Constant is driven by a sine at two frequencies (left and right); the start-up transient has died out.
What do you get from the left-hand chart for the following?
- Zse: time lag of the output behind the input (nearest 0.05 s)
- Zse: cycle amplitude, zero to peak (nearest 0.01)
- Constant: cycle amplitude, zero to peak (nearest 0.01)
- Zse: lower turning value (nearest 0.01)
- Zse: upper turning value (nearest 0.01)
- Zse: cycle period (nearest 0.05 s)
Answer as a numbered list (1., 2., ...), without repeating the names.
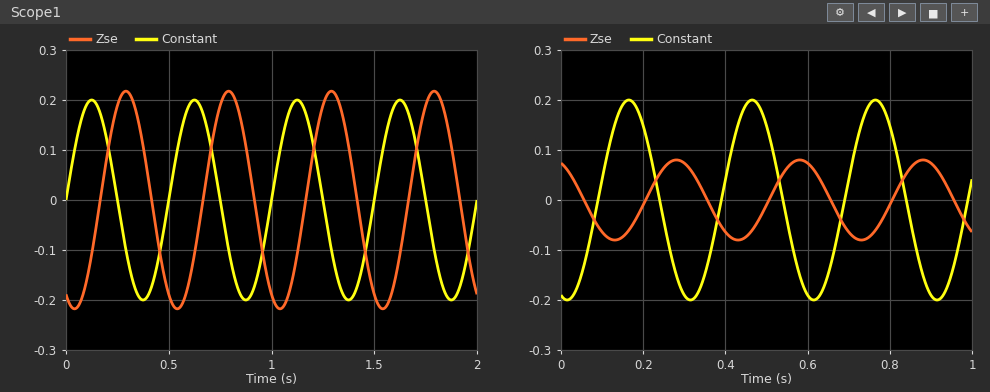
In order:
1. 0.15 s
2. 0.22
3. 0.20
4. -0.22
5. 0.22
6. 0.50 s
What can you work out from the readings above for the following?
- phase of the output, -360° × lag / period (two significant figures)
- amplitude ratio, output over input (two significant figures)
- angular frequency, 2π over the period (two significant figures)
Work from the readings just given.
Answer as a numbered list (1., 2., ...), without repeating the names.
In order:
1. -110°
2. 1.1
3. 13 rad/s
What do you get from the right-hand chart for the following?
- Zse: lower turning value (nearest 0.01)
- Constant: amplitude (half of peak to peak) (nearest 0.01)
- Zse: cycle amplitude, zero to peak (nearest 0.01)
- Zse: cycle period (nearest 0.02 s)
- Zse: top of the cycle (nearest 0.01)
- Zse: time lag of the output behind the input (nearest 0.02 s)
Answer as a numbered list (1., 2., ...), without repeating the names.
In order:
1. -0.08
2. 0.20
3. 0.08
4. 0.30 s
5. 0.08
6. 0.12 s
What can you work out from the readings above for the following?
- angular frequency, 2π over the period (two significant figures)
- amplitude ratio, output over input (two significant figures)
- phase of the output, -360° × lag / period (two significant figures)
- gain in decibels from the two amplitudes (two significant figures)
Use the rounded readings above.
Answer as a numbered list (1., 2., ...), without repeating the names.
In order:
1. 21 rad/s
2. 0.40
3. -140°
4. -8.0 dB
